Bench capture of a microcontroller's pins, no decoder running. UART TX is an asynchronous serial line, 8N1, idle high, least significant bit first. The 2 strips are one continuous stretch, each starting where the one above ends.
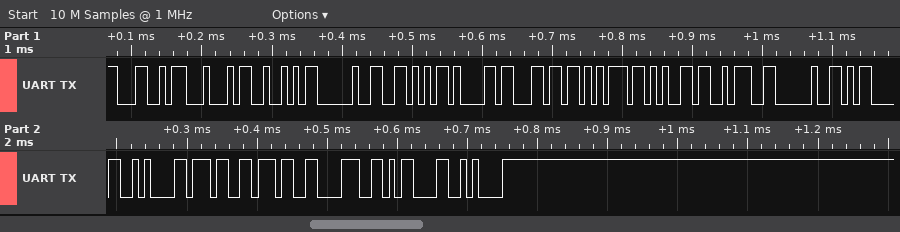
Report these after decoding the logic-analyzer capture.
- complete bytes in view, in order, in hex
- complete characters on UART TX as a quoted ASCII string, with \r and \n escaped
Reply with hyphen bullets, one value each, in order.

- 0x4C 0x44 0x52 0x20 0x56 0x61 0x6C 0x75 0x65 0x3A 0x20 0x0D 0x0A 0x37 0x37 0x38 0x0D 0x0A
- "LDR Value: \r\n778\r\n"
